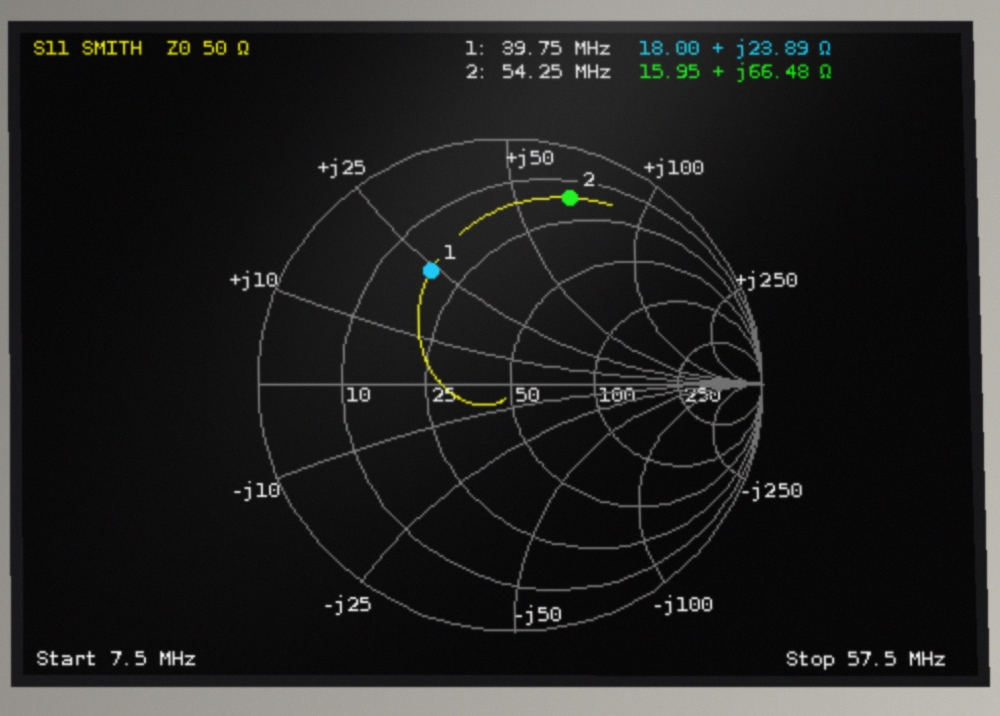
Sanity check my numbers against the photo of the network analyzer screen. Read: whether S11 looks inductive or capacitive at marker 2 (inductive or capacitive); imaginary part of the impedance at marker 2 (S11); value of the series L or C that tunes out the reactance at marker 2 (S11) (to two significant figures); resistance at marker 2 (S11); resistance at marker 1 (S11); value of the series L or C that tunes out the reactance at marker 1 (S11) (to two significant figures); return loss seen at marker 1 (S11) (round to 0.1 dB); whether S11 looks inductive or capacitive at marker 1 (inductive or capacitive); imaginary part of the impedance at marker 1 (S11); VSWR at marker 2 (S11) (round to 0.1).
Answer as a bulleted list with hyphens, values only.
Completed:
- inductive
- +66.48 Ω
- 44 pF
- 15.95 Ω
- 18.00 Ω
- 170 pF
- 5.1 dB
- inductive
- +23.89 Ω
- 8.9
